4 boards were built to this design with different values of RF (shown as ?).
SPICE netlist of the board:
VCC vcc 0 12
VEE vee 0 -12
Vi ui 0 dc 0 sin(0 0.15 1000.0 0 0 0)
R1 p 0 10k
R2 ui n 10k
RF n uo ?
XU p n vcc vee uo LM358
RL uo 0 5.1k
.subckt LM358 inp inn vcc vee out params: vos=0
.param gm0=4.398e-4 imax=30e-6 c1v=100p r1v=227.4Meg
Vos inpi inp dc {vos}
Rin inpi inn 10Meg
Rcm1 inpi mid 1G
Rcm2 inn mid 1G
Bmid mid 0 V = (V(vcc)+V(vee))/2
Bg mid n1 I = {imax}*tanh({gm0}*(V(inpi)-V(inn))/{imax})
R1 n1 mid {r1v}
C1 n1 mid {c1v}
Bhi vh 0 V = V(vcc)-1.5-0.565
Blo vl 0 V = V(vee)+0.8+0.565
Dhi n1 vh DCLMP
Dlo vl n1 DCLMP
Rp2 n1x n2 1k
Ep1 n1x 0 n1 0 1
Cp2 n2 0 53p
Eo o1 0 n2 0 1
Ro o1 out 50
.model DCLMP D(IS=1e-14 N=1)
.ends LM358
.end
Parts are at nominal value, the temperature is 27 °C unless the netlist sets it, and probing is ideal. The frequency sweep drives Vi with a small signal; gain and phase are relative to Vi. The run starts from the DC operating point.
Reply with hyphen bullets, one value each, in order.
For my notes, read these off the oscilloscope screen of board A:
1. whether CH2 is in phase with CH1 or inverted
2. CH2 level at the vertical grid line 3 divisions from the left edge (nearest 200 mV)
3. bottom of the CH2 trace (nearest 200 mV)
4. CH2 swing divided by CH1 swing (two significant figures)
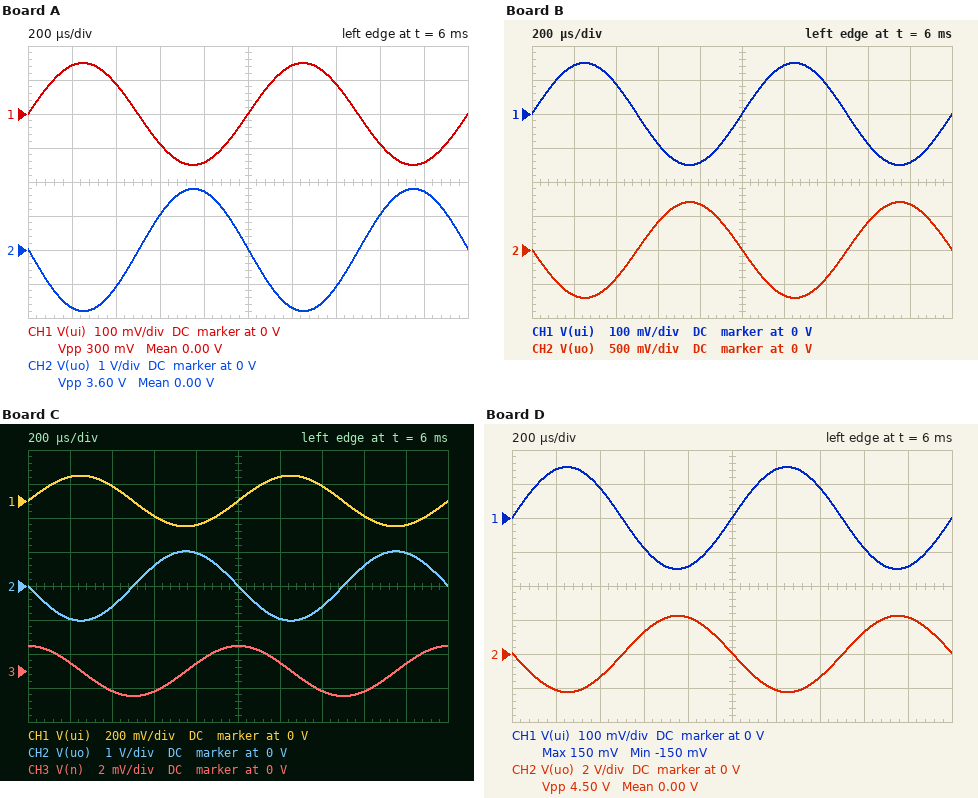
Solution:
- inverted
- 1.0 V
- -1.8 V
- 12
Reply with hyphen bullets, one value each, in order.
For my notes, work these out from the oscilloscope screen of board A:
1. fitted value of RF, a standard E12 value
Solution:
- 120 kΩ
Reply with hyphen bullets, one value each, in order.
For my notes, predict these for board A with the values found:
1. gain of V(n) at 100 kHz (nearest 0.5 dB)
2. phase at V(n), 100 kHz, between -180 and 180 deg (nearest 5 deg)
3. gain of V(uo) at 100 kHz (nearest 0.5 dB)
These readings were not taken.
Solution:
- -1.5 dB
- 30 deg
- 15.0 dB
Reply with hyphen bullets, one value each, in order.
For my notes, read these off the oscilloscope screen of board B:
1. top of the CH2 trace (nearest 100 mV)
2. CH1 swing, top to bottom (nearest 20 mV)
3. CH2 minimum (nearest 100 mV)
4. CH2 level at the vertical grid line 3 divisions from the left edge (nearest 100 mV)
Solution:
- 700 mV
- 300 mV
- -700 mV
- 400 mV
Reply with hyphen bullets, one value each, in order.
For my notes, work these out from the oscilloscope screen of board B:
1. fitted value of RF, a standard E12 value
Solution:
- 47 kΩ
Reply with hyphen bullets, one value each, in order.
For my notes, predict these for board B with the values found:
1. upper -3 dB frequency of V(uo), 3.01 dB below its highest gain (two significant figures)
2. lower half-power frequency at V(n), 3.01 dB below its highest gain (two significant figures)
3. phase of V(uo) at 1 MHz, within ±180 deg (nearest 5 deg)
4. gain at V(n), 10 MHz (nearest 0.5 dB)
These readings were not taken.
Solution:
- 130 kHz
- 120 kHz
- 80 deg
- -1.5 dB
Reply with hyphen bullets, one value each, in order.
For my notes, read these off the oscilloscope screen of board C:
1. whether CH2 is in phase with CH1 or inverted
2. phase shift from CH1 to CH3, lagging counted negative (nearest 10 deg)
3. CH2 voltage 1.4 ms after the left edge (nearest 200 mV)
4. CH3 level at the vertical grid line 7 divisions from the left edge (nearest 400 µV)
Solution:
- inverted
- 90 deg
- -600 mV
- -1.2 mV
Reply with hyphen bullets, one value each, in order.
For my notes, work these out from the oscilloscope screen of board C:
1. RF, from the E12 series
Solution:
- 68 kΩ
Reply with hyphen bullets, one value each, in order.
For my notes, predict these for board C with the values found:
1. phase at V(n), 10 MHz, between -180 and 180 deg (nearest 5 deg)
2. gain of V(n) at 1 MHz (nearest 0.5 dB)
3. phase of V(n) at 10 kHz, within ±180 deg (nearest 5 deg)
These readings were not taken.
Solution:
- 0 deg
- -1.0 dB
- 85 deg
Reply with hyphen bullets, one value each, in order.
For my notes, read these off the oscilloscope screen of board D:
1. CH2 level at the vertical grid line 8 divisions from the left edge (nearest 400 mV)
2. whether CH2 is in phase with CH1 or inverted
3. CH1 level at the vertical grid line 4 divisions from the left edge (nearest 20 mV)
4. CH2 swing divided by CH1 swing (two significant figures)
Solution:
- 1.2 V
- inverted
- -140 mV
- 15
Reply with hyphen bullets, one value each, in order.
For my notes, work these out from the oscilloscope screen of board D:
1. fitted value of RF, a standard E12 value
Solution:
- 150 kΩ
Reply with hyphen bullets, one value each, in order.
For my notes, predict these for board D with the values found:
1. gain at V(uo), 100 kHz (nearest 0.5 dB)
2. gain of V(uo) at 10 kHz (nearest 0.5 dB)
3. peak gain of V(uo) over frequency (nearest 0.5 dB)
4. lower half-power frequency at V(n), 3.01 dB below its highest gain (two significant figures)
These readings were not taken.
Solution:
- 15.5 dB
- 23.5 dB
- 23.5 dB
- 44 kHz
